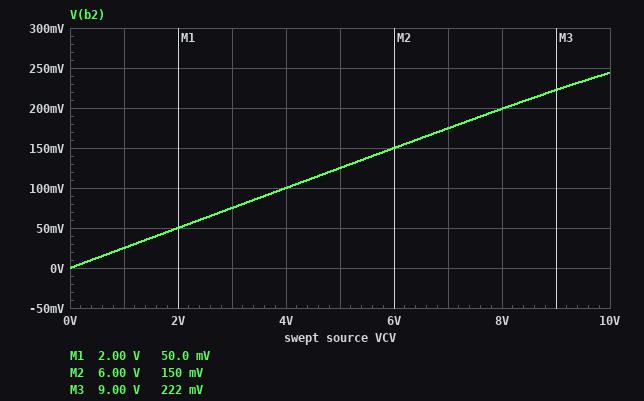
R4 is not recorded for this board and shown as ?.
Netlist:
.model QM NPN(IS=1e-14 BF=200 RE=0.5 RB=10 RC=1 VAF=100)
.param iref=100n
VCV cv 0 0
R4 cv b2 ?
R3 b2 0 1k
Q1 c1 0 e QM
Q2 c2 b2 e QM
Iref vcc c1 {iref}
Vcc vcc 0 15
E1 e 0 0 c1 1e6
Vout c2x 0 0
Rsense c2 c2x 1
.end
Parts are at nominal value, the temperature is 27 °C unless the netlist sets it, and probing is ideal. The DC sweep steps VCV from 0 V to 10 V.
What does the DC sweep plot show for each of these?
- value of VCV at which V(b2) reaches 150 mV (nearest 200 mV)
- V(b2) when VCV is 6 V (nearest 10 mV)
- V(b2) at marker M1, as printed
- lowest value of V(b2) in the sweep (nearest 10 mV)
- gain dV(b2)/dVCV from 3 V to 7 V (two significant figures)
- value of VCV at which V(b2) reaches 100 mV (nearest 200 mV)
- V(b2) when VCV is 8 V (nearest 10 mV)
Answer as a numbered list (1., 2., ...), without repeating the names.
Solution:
1. 6.0 V
2. 150 mV
3. 50.0 mV
4. 0 V
5. 0.025 V/V
6. 4.0 V
7. 200 mV
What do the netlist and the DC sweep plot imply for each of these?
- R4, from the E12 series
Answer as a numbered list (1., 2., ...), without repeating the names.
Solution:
1. 39 kΩ
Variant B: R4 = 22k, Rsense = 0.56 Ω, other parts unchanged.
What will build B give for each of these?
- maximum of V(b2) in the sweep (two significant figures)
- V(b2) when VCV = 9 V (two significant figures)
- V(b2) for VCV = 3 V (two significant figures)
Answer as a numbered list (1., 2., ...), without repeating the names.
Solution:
1. 330 mV
2. 320 mV
3. 130 mV
